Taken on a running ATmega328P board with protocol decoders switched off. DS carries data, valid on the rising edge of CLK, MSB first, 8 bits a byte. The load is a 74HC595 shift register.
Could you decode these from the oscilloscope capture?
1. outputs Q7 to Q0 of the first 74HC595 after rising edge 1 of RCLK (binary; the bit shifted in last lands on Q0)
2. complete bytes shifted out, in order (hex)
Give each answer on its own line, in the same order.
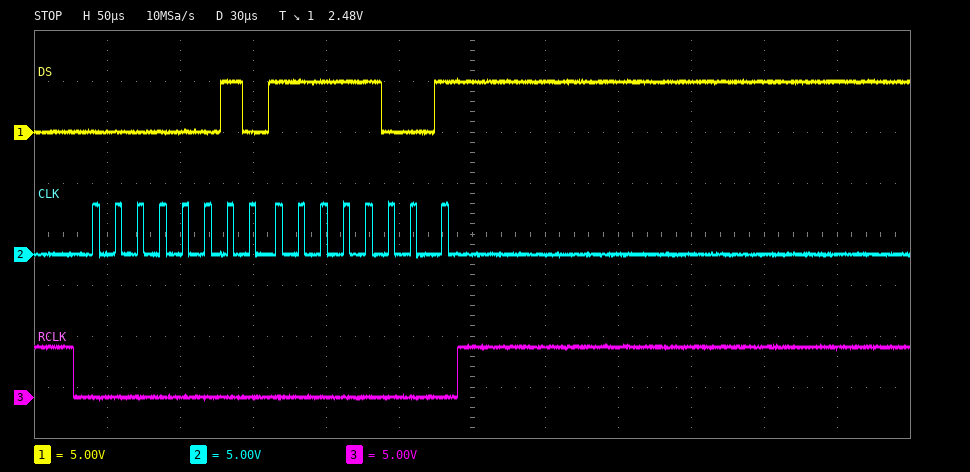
11111001
02 F9
